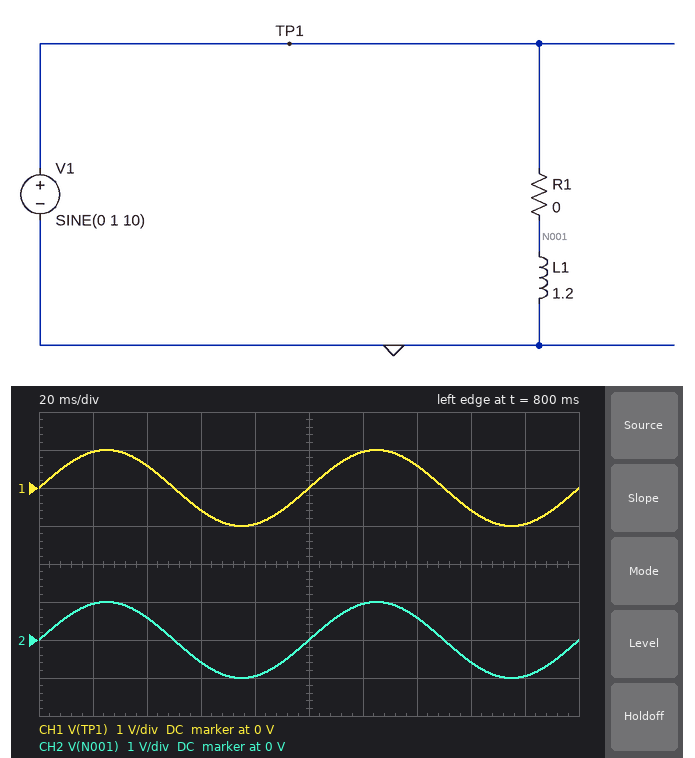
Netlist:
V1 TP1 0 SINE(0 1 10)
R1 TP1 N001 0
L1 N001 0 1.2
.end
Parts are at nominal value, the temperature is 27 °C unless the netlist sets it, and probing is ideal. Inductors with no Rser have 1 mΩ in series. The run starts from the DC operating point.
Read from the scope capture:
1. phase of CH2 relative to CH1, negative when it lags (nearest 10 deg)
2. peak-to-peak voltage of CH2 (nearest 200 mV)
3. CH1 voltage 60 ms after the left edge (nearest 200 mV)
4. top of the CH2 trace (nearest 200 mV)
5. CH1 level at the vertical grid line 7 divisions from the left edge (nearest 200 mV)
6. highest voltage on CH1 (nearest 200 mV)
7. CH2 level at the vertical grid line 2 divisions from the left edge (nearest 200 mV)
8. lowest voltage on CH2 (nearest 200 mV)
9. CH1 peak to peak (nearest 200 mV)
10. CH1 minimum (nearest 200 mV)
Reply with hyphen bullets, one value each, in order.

- 0 deg
- 2.0 V
- -600 mV
- 1.0 V
- 600 mV
- 1.0 V
- 600 mV
- -1.0 V
- 2.0 V
- -1.0 V
